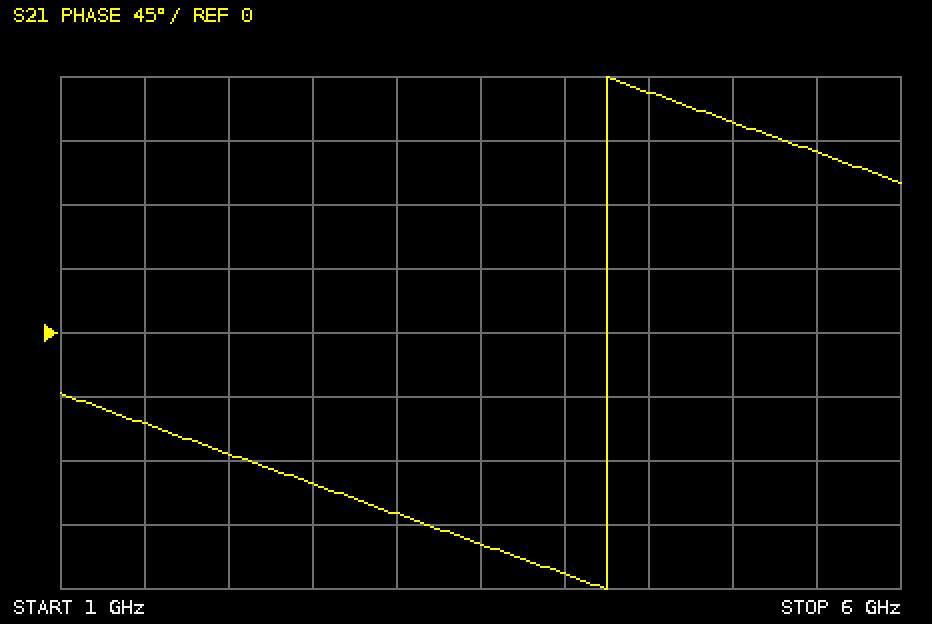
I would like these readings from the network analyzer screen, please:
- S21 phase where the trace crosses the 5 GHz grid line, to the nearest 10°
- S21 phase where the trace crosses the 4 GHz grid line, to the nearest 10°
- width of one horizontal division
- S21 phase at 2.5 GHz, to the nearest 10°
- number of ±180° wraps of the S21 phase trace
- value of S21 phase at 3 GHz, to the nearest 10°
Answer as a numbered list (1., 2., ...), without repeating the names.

1. 150°
2. -170°
3. 500 MHz
4. -110°
5. 1
6. -130°
